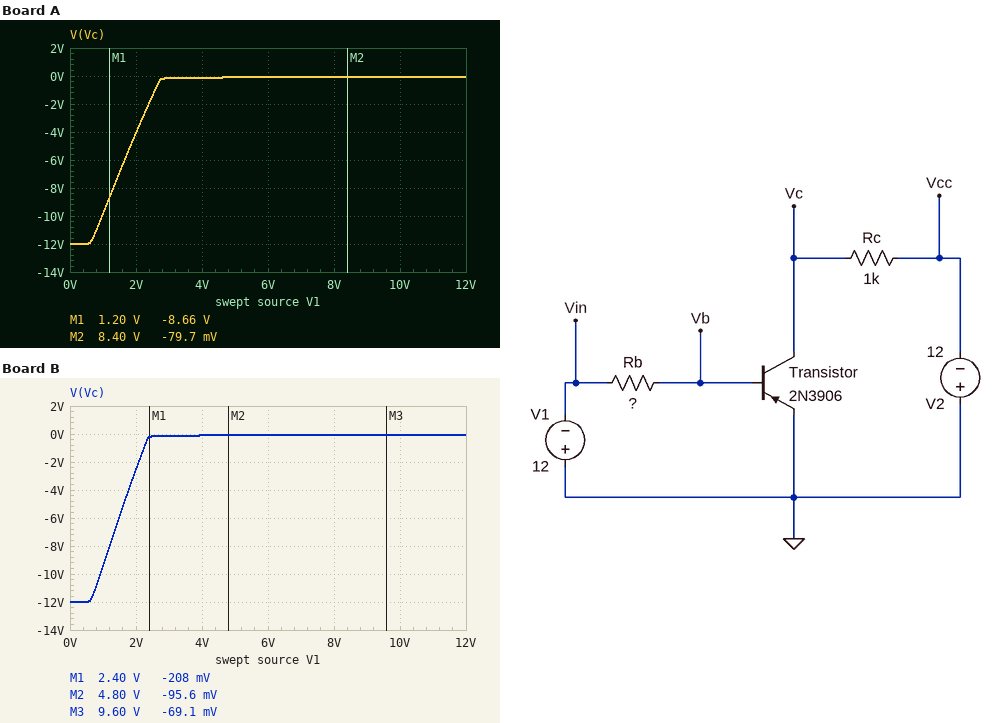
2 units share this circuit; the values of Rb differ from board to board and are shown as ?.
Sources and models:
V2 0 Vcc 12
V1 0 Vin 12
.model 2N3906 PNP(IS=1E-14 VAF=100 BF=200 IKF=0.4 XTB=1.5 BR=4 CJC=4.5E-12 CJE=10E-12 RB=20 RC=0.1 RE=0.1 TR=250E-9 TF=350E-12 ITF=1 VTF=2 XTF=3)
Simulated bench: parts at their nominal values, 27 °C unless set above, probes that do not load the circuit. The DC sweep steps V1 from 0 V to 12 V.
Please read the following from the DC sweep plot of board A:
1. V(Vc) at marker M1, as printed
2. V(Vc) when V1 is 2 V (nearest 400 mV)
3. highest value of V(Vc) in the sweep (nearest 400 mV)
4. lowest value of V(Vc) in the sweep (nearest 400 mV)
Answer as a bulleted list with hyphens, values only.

- -8.66 V
- -4.0 V
- 0 V
- -12.0 V
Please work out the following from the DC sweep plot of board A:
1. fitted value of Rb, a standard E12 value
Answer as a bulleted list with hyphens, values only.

- 33 kΩ
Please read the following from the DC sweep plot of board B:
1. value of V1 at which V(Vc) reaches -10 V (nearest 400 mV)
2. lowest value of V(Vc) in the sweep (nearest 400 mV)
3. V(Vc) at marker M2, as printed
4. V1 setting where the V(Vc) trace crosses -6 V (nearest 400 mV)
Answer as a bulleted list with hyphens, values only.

- 800 mV
- -12.0 V
- -95.6 mV
- 1.6 V
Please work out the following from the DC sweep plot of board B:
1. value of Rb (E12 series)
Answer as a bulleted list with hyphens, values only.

- 27 kΩ
